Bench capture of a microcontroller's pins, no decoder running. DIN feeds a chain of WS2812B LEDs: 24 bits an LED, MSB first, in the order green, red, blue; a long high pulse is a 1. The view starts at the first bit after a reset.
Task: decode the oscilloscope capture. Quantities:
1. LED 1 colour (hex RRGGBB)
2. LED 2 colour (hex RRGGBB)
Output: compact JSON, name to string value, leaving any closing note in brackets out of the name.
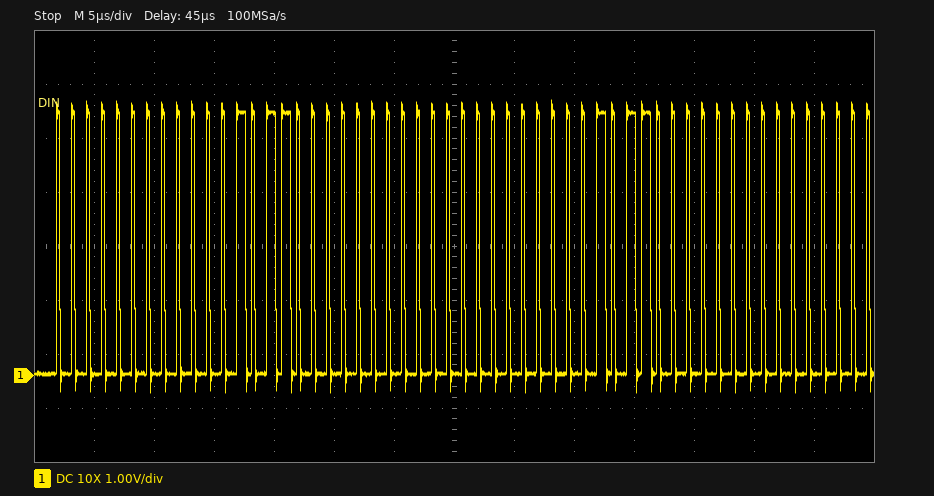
{"LED 1 colour": "#0B0000", "LED 2 colour": "#0B0000"}
